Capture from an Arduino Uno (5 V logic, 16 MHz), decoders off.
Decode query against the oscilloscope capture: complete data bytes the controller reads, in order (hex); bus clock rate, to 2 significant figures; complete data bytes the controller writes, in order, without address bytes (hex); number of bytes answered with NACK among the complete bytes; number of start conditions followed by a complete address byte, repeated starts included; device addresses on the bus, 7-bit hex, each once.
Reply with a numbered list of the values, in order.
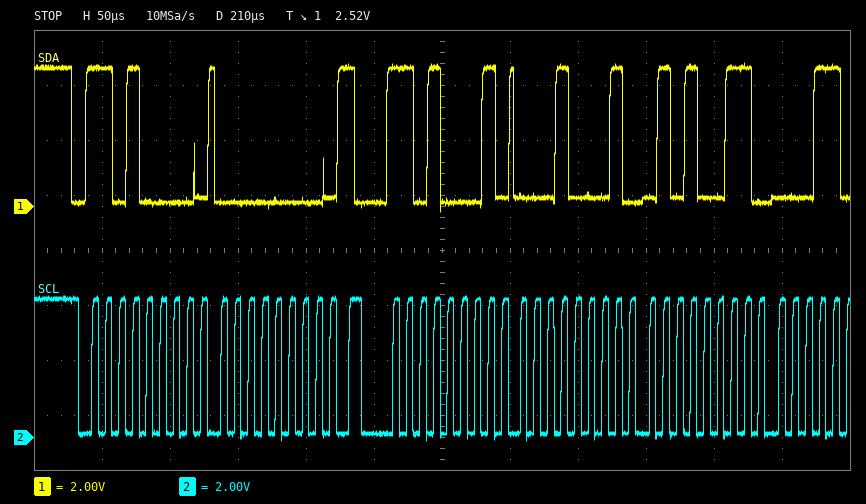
1. 11 53
2. 100 kHz
3. 00
4. 0
5. 2
6. 0x68
